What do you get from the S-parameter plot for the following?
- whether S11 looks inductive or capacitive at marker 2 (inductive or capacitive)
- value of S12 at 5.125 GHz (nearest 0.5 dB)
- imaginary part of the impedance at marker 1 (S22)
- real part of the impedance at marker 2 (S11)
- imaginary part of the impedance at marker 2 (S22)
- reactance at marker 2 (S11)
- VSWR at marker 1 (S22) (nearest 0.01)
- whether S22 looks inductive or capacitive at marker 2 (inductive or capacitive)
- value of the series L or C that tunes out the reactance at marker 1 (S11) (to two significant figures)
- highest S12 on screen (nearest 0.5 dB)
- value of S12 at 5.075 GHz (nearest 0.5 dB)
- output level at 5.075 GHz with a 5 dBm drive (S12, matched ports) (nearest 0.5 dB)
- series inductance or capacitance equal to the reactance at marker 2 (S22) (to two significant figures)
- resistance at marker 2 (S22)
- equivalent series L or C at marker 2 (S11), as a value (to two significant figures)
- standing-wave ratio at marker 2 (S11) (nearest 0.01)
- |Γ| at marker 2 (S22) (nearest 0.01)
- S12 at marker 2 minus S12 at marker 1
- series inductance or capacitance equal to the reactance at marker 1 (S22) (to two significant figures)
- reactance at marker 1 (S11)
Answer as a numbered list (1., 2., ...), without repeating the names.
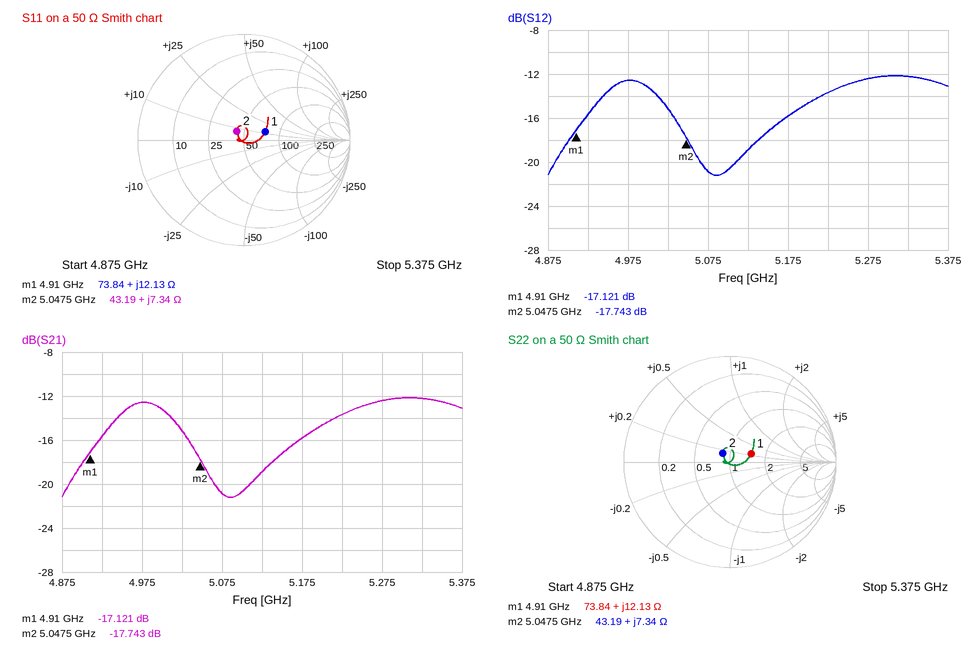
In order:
1. inductive
2. -19.0 dB
3. +12.13 Ω
4. 43.19 Ω
5. +7.34 Ω
6. +7.34 Ω
7. 1.55
8. inductive
9. 2.7 pF
10. -12.0 dB
11. -21.0 dB
12. -16.0 dBm
13. 230 pH
14. 43.19 Ω
15. 230 pH
16. 1.24
17. 0.11
18. -0.622 dB
19. 390 pH
20. +12.13 Ω
